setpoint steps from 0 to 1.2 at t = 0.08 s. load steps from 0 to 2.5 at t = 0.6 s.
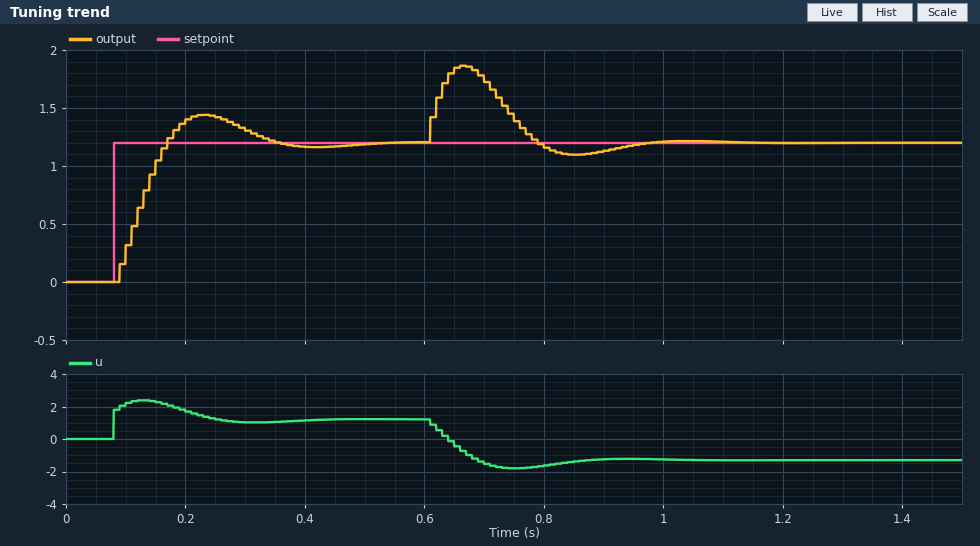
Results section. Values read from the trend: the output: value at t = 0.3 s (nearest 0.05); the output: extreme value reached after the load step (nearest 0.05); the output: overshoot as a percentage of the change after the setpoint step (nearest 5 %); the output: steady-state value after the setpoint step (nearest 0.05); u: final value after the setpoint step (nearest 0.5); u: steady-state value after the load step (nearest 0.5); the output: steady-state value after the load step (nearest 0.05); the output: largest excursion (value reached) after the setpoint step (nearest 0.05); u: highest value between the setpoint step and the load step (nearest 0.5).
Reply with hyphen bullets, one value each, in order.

- 1.30
- 1.85
- 20 %
- 1.20
- 1.0
- -1.5
- 1.20
- 1.45
- 2.5
